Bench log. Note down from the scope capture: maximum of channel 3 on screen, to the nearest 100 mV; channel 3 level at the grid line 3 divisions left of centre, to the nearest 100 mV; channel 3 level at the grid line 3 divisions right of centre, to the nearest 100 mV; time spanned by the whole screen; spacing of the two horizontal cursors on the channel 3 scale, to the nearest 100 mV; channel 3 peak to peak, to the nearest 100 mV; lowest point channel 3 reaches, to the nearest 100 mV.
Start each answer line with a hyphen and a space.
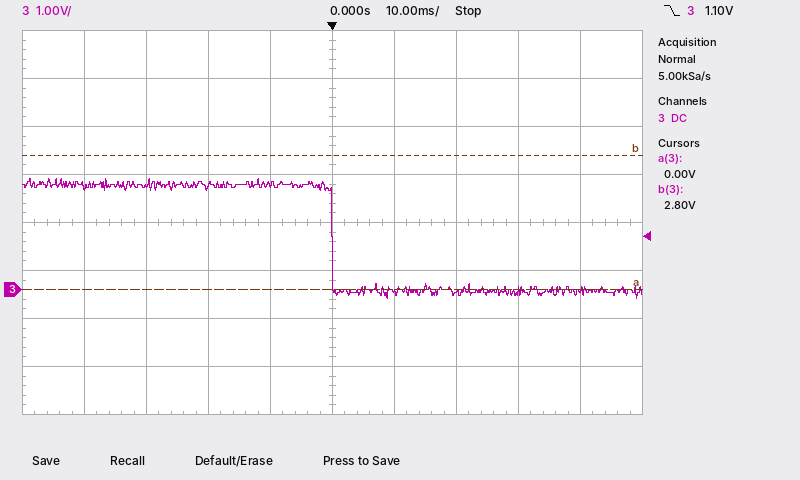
- 2.3 V
- 2.2 V
- 0.0 V
- 100 ms
- 2.8 V
- 2.5 V
- -200 mV
